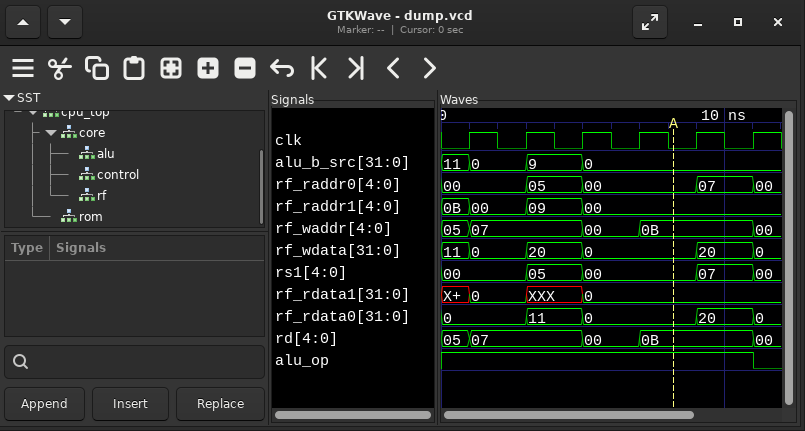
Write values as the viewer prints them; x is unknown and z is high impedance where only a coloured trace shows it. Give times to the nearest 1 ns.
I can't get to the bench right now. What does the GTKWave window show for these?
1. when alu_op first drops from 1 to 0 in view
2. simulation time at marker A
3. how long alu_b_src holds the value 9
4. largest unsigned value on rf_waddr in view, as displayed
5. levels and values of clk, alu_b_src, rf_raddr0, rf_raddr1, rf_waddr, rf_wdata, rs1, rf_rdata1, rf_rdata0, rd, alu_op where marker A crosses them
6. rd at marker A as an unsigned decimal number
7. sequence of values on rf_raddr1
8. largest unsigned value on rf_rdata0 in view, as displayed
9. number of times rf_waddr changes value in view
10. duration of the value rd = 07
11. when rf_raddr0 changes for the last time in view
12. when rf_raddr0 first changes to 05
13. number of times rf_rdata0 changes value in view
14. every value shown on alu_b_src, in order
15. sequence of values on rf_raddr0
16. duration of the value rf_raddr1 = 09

11 ns
8 ns
2 ns
0B
clk=0, alu_b_src=0, rf_raddr0=00, rf_raddr1=00, rf_waddr=0B, rf_wdata=0, rs1=00, rf_rdata1=0, rf_rdata0=0, rd=0B, alu_op=1
11
0B, 00, 09, 00
20
4
4 ns
11 ns
3 ns
4
11, 0, 9, 0
00, 05, 00, 07, 00
2 ns
